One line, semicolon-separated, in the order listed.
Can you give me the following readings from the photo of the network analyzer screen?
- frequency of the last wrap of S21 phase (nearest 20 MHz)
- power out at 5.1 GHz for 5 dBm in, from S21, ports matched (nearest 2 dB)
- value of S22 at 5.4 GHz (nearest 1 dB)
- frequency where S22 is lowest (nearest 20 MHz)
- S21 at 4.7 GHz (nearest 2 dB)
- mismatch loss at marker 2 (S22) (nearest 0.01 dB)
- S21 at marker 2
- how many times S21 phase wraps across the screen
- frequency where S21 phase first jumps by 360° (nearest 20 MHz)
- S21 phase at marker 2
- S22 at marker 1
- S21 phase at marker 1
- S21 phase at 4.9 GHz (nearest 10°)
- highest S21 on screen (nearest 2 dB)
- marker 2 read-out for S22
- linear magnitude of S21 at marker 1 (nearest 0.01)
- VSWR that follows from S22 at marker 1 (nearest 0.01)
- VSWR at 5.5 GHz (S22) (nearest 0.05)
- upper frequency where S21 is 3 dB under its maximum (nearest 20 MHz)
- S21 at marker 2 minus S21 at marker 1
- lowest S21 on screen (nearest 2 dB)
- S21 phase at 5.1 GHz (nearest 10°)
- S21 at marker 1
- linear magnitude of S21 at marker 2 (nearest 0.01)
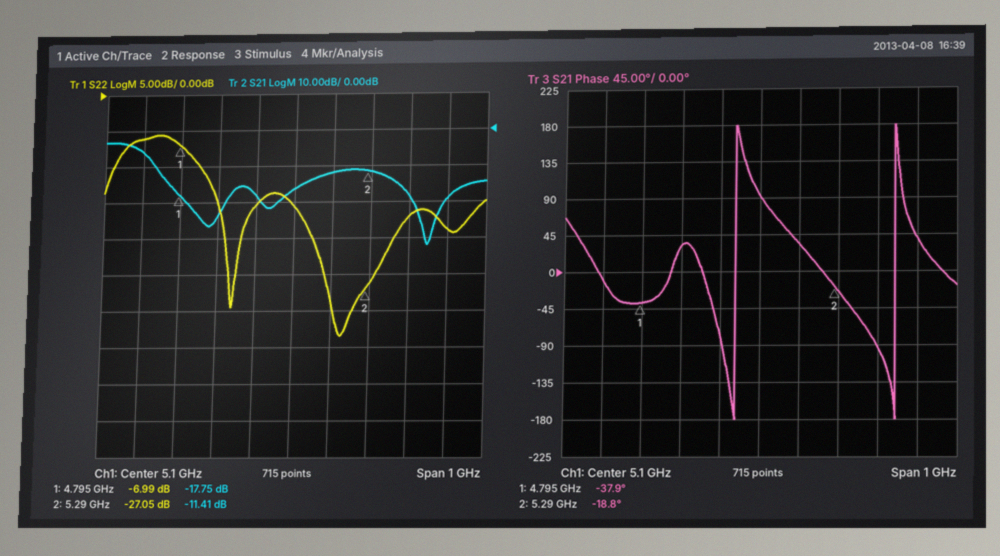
5.44 GHz; -12 dBm; -17 dB; 5.22 GHz; -6 dB; 0.01 dB; -11.41 dB; 2; 5.04 GHz; -18.8°; -6.99 dB; -37.9°; 30°; -4 dB; -27.05 dB; 0.13; 2.62; 1.25; 4.70 GHz; 6.34 dB; -32 dB; 90°; -17.75 dB; 0.27
